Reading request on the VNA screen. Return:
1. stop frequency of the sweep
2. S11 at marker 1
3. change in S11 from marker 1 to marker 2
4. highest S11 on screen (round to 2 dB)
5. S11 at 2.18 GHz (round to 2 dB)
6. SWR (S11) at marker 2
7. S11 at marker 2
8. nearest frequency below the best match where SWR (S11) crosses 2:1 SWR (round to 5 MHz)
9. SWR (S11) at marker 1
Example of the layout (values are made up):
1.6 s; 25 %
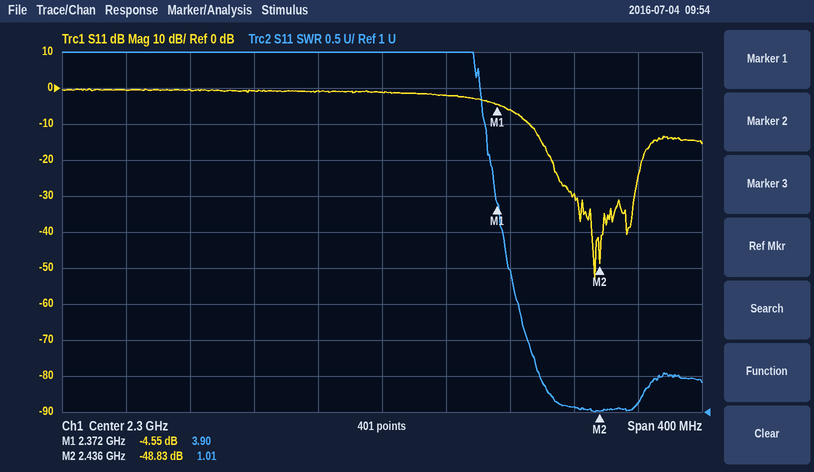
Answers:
2.5 GHz; -4.55 dB; -44.28 dB; 0 dB; 0 dB; 1.01; -48.83 dB; 2.390 GHz; 3.90
